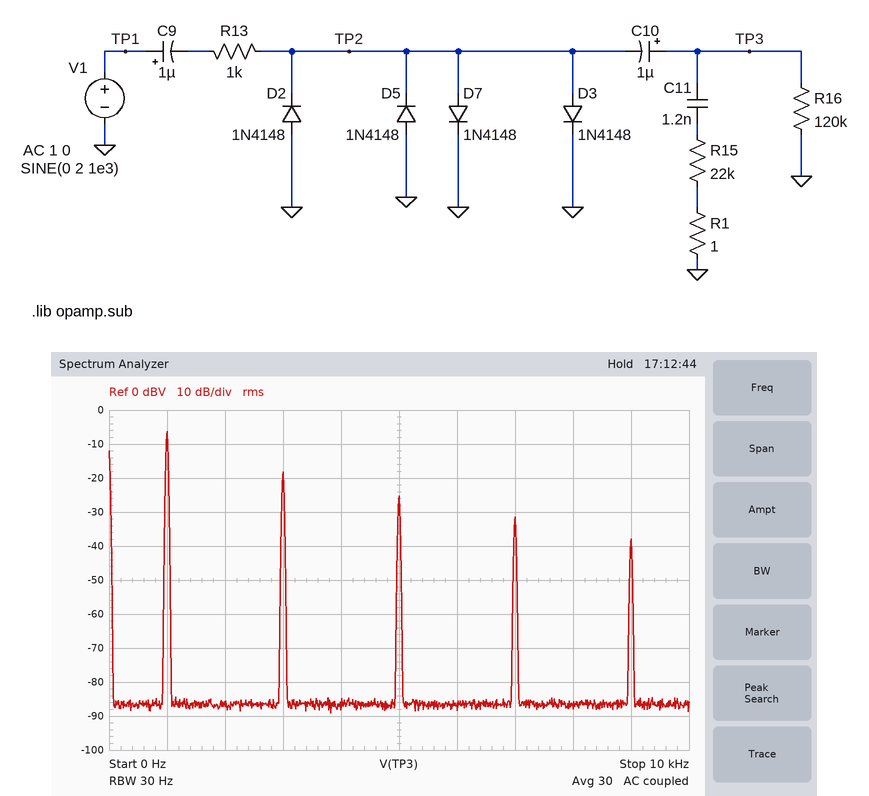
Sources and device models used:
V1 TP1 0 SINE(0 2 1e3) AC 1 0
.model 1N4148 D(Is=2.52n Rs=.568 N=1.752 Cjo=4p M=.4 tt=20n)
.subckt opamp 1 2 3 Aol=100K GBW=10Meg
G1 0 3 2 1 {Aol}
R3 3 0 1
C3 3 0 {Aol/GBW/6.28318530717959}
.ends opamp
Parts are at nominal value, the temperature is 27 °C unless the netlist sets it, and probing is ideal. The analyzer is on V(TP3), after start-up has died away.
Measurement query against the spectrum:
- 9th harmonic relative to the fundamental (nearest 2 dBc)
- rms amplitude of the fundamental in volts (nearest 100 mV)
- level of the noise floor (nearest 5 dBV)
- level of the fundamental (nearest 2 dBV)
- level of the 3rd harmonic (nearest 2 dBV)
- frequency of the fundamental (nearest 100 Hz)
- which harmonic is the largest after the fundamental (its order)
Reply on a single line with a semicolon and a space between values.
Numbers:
-32 dBc; 500 mV; -85 dBV; -6 dBV; -18 dBV; 1.0 kHz; 3
